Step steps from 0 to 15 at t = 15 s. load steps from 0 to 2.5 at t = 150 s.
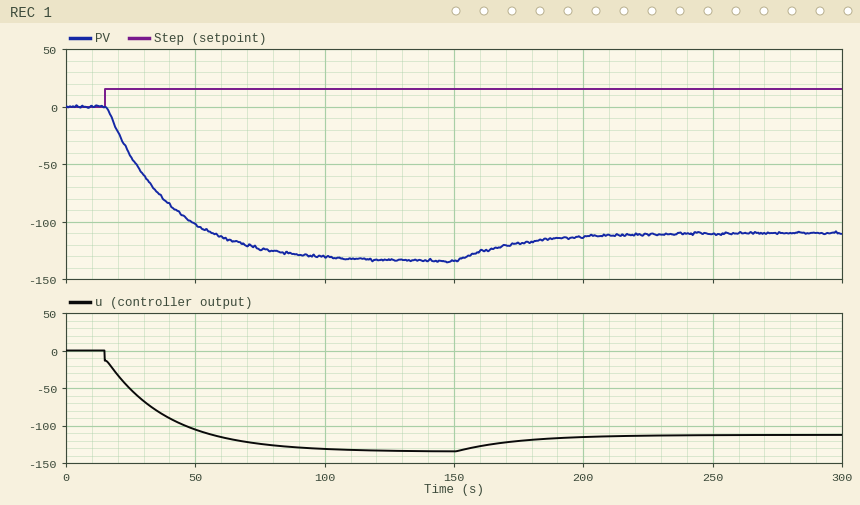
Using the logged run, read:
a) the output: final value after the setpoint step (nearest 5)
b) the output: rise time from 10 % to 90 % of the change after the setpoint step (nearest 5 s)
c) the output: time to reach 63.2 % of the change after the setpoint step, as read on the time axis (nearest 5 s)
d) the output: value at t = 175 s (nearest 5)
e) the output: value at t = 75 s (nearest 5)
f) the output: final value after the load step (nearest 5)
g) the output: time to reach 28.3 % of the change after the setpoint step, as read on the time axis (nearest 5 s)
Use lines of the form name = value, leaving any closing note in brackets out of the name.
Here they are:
the output: final value after the setpoint step = -135
the output: rise time from 10 % to 90 % of the change after the setpoint step = 55 s
the output: time to reach 63.2 % of the change after the setpoint step, as read on the time axis = 40 s
the output: value at t = 175 s = -120
the output: value at t = 75 s = -125
the output: final value after the load step = -110
the output: time to reach 28.3 % of the change after the setpoint step, as read on the time axis = 25 s
